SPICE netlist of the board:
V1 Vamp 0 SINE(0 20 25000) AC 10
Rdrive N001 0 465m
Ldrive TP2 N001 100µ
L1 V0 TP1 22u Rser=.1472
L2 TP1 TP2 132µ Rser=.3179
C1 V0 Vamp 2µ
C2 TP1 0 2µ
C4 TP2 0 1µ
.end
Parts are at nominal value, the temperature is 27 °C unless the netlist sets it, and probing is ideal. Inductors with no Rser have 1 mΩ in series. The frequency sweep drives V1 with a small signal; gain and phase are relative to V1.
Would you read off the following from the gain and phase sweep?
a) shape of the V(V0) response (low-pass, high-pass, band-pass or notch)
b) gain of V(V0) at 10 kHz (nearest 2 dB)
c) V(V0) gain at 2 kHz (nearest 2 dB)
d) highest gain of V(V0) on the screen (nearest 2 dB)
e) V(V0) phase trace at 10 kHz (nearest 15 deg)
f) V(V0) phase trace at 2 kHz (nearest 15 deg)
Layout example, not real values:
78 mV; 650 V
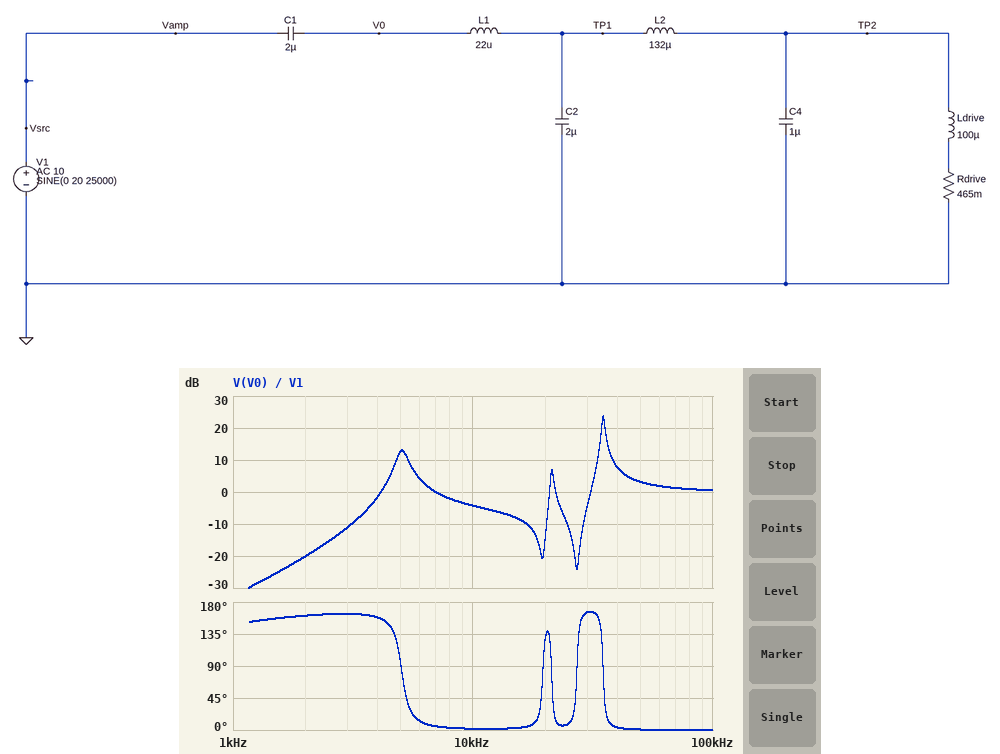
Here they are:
high-pass; -4 dB; -20 dB; 24 dB; 0 deg; 165 deg
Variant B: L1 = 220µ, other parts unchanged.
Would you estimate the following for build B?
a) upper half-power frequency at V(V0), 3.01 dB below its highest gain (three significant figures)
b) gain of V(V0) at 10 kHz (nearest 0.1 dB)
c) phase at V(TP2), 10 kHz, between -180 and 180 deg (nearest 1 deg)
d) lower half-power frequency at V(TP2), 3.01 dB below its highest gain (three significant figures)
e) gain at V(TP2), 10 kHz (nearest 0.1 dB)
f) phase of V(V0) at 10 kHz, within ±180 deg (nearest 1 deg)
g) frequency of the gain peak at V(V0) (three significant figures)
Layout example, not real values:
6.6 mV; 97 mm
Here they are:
11.8 kHz; -17.9 dB; -6 deg; 11.5 kHz; -0.3 dB; 86 deg; 11.7 kHz
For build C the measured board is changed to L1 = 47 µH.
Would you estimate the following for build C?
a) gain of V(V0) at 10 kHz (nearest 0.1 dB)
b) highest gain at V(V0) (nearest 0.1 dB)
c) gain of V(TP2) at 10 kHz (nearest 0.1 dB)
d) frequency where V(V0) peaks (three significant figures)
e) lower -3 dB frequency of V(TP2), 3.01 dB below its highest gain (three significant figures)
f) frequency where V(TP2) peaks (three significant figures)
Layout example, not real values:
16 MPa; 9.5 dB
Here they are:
-4.8 dB; 22.7 dB; -7.8 dB; 25.5 kHz; 19.9 kHz; 20.2 kHz
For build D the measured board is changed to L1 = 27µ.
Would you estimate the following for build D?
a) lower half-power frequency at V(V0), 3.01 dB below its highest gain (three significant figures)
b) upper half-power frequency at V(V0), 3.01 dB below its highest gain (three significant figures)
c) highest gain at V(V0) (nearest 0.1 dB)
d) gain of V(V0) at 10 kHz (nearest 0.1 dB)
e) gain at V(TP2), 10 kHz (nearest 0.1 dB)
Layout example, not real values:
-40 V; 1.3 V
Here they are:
31.4 kHz; 32.2 kHz; 24.2 dB; -4.4 dB; -8.3 dB
